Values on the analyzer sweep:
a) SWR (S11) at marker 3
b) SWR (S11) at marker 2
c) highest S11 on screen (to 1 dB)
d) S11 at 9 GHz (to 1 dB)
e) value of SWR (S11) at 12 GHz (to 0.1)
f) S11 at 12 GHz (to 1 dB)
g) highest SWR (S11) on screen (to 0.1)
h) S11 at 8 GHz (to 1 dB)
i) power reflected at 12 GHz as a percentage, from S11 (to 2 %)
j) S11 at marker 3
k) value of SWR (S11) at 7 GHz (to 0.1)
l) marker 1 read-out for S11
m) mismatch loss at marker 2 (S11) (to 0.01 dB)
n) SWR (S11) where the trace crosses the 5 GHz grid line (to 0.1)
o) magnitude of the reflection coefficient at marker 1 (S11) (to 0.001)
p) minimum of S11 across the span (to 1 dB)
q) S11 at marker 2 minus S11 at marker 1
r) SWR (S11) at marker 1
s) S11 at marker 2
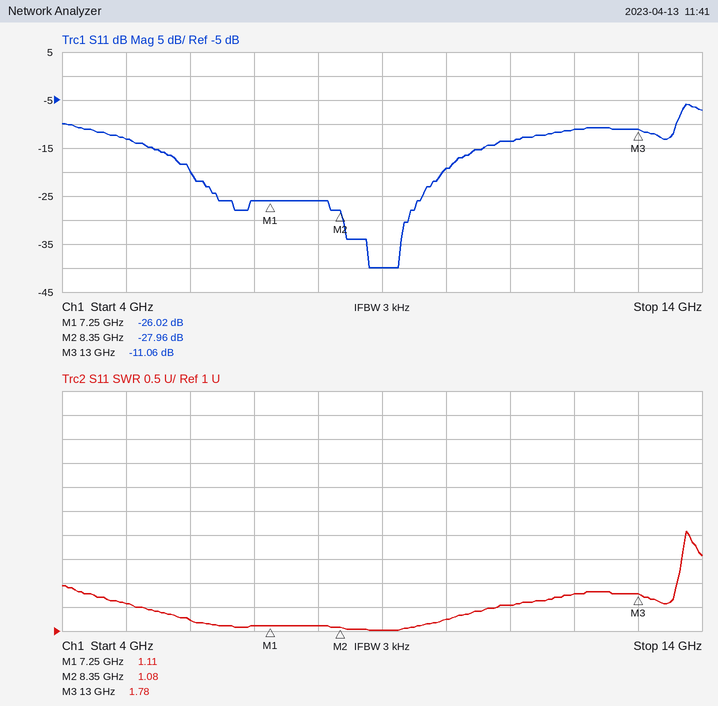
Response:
1.78
1.08
-6 dB
-40 dB
1.8
-11 dB
3.1
-26 dB
8 %
-11.06 dB
1.1
-26.02 dB
0.01 dB
1.6
0.050
-40 dB
-1.94 dB
1.11
-27.96 dB
